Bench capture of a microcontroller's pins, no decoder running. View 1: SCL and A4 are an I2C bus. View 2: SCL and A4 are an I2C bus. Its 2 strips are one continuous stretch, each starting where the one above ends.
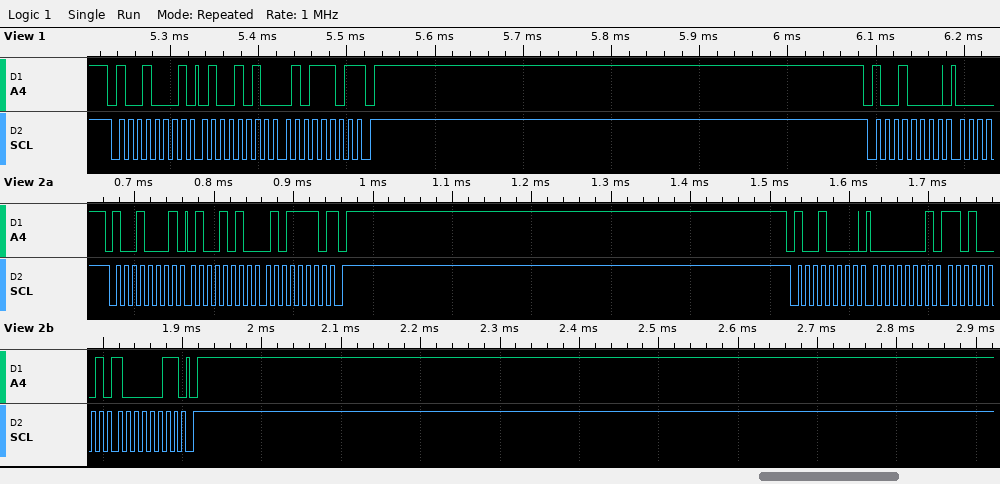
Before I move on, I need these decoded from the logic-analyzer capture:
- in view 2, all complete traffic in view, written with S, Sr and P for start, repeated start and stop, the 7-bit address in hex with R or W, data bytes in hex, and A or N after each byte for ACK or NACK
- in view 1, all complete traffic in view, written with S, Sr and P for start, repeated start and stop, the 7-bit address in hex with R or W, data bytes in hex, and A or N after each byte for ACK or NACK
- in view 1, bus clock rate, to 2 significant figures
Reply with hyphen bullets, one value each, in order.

- S 48R A 4A A 5E N P S 48W A 01 A D1 A 83 A P
- S 48R A 4A A 5D N P S 48W A
- 100 kHz
